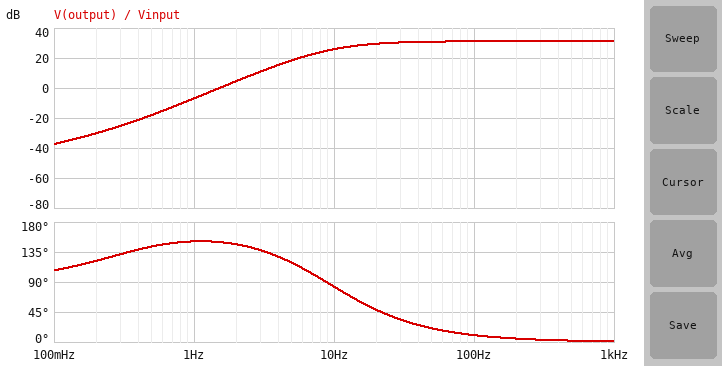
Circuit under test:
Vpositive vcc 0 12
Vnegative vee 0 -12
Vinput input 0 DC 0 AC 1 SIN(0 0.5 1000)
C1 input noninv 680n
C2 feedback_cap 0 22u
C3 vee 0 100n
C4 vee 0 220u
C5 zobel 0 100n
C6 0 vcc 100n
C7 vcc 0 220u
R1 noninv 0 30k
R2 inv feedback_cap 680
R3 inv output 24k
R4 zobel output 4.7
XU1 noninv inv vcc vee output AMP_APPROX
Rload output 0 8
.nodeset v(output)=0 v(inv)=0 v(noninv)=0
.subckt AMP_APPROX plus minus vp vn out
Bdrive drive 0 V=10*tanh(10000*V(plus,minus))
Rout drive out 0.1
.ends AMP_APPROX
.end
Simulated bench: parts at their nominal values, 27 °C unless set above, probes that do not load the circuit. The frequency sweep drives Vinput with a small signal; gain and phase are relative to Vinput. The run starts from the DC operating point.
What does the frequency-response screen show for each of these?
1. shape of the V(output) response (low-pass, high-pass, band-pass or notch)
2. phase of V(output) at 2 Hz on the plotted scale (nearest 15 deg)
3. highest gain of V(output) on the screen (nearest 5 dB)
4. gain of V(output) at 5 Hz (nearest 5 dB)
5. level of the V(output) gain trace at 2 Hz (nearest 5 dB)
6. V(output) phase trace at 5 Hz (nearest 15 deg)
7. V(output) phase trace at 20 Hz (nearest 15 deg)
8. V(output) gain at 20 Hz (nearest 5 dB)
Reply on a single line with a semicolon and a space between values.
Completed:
high-pass; 150 deg; 30 dB; 20 dB; 5 dB; 120 deg; 45 deg; 30 dB
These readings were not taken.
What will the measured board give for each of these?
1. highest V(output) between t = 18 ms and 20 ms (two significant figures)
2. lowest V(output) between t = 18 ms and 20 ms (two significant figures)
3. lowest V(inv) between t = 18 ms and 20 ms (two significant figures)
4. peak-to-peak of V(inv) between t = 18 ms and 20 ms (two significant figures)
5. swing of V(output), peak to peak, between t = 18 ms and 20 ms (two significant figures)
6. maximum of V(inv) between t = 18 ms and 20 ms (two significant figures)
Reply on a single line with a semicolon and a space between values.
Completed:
9.9 V; -9.9 V; -270 mV; 550 mV; 20 V; 280 mV
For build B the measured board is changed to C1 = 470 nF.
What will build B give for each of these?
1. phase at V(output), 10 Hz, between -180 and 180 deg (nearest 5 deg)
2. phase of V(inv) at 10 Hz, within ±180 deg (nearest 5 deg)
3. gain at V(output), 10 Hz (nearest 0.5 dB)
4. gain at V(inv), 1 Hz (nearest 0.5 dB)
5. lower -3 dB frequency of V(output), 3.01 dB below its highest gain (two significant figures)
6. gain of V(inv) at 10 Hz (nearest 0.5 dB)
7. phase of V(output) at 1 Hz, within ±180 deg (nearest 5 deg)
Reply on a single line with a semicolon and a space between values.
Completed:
95 deg; 50 deg; 24.5 dB; -21.0 dB; 17 Hz; -3.5 dB; 155 deg
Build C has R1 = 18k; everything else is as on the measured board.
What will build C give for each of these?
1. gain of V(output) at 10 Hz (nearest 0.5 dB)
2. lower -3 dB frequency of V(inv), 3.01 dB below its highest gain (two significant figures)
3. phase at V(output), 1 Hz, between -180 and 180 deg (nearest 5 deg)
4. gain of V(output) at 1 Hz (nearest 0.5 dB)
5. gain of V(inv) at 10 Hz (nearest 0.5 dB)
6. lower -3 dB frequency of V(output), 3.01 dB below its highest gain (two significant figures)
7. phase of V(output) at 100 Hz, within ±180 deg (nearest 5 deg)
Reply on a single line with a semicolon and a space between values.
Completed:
23.5 dB; 13 Hz; 155 deg; -11.5 dB; -4.5 dB; 18 Hz; 15 deg
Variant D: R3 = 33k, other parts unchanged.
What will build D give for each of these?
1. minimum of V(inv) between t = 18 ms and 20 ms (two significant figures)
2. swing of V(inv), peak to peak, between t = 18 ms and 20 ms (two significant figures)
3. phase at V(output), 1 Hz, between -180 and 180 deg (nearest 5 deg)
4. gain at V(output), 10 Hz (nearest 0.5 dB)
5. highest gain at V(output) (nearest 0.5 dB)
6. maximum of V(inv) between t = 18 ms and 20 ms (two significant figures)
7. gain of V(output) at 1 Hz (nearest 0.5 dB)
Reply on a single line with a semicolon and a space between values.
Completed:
-200 mV; 400 mV; 155 deg; 28.5 dB; 34.0 dB; 200 mV; -4.5 dB
